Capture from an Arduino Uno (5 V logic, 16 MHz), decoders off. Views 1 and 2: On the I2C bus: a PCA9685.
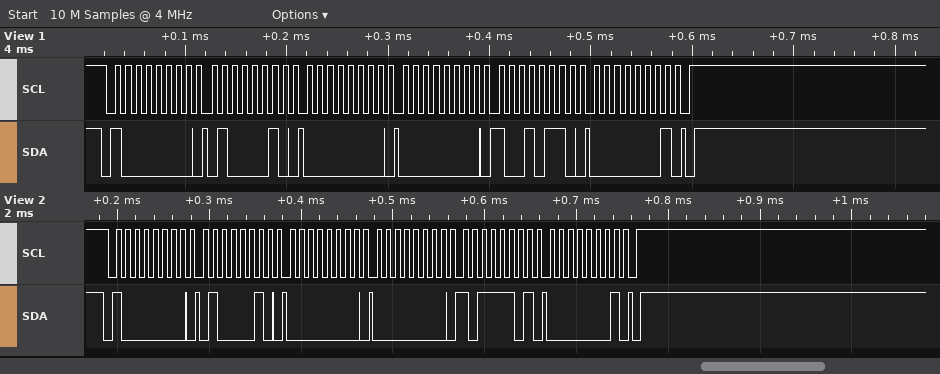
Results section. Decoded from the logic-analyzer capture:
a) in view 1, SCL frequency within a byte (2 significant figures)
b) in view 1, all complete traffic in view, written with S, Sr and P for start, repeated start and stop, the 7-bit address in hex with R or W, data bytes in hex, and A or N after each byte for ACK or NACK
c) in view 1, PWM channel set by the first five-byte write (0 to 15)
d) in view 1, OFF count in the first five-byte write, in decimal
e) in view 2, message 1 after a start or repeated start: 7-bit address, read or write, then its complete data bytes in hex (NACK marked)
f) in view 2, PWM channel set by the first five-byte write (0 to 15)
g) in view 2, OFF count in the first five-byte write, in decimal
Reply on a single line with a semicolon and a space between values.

100 kHz; S 40W A 42 A 00 A 00 A 96 A 01 A P; 15; 406; 0x40 write: 42 00 00 BD 01; 15; 445
